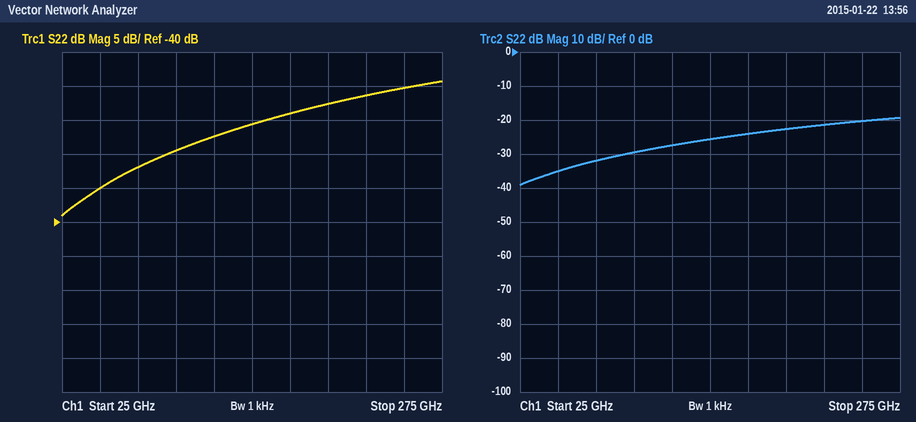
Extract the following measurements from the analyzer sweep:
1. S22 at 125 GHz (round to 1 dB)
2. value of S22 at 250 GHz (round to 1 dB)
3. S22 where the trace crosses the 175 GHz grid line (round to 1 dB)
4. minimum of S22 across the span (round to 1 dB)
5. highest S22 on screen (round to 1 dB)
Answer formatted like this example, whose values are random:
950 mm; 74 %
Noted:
-27 dB; -20 dB; -24 dB; -39 dB; -19 dB
